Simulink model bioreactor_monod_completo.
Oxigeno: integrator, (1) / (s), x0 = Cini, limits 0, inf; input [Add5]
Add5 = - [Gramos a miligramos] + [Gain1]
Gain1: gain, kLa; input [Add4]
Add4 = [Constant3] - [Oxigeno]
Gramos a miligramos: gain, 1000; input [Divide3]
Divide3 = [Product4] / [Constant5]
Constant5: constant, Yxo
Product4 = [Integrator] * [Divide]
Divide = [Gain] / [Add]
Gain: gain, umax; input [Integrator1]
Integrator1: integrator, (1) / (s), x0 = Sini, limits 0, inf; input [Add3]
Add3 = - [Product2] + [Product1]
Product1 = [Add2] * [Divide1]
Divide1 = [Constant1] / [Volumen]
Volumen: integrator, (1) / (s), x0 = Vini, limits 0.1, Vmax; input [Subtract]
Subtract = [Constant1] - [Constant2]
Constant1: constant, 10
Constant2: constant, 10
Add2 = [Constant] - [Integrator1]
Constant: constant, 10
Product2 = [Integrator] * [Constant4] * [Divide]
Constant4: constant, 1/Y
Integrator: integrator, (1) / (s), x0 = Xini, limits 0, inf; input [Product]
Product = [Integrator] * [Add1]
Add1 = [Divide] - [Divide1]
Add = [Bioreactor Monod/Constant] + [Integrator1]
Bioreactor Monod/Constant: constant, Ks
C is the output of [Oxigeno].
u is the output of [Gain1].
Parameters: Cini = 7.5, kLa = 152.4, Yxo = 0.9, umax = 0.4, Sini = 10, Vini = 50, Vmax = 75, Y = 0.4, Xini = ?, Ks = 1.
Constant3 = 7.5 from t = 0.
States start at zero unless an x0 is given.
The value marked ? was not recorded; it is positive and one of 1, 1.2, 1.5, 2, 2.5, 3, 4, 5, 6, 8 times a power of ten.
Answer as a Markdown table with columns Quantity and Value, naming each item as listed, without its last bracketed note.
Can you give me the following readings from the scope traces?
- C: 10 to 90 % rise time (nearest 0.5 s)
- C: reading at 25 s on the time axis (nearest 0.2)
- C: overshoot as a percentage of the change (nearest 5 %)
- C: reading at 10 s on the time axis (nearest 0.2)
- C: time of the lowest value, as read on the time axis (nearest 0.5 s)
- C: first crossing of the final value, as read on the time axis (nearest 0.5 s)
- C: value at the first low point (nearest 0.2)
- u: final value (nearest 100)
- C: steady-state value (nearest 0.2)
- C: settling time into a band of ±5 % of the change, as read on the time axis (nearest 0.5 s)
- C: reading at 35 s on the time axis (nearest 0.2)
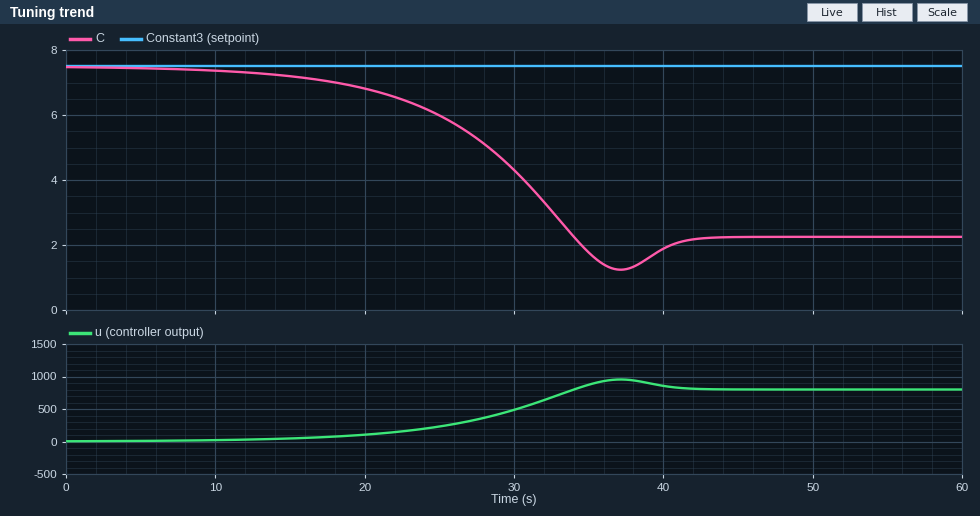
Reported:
| Quantity | Value |
|---|---|
| C: 10 to 90 % rise time | 14.5 s |
| C: reading at 25 s on the time axis | 6.0 |
| C: overshoot as a percentage of the change | 20 % |
| C: reading at 10 s on the time axis | 7.4 |
| C: time of the lowest value, as read on the time axis | 37.0 s |
| C: first crossing of the final value, as read on the time axis | 34.0 s |
| C: value at the first low point | 1.2 |
| u: final value | 800 |
| C: steady-state value | 2.2 |
| C: settling time into a band of ±5 % of the change, as read on the time axis | 40.5 s |
| C: reading at 35 s on the time axis | 1.8 |
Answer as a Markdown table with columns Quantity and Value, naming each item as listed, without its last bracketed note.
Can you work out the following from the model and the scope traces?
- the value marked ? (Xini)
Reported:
| Quantity | Value |
|---|---|
| the value marked ? | 0.01 |
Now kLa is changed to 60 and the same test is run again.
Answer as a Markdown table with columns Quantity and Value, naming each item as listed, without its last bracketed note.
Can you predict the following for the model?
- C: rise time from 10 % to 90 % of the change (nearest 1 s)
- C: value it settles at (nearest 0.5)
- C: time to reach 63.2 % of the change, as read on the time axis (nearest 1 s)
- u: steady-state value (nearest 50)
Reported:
| Quantity | Value |
|---|---|
| C: rise time from 10 % to 90 % of the change | 14 s |
| C: value it settles at | 0.0 |
| C: time to reach 63.2 % of the change, as read on the time axis | 26 s |
| u: steady-state value | 450 |
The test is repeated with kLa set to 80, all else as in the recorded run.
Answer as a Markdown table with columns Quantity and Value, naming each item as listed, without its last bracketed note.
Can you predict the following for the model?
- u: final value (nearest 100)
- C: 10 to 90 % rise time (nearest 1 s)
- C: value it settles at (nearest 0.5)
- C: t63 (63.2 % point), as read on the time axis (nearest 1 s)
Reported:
| Quantity | Value |
|---|---|
| u: final value | 600 |
| C: 10 to 90 % rise time | 14 s |
| C: value it settles at | 0.0 |
| C: t63 (63.2 % point), as read on the time axis | 28 s |
